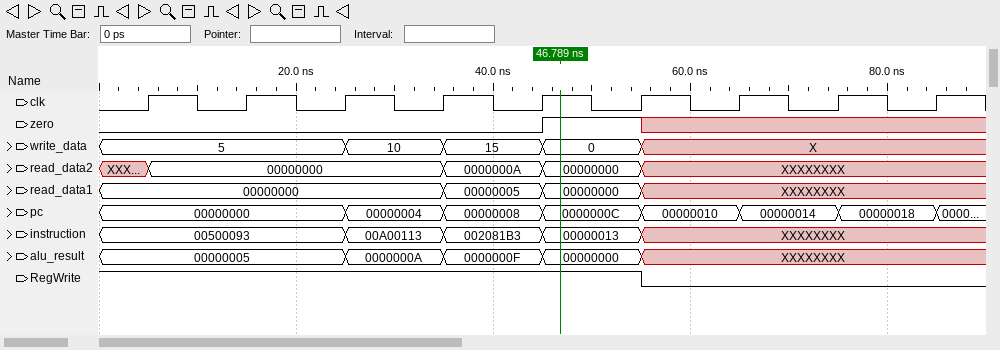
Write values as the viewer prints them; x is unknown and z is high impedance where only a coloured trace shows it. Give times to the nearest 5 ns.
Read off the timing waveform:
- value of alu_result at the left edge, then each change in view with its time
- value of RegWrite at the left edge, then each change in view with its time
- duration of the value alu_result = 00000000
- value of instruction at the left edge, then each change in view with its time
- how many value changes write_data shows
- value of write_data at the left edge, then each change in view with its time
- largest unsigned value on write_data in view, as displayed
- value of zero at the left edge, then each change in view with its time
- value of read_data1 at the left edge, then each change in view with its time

00000005, 0000000A at 25 ns, 0000000F at 35 ns, 00000000 at 45 ns, XXXXXXXX at 55 ns
1, 0 at 55 ns
10 ns
00500093, 00A00113 at 25 ns, 002081B3 at 35 ns, 00000013 at 45 ns, XXXXXXXX at 55 ns
4
5, 10 at 25 ns, 15 at 35 ns, 0 at 45 ns, X at 55 ns
15
0, 1 at 45 ns, x at 55 ns
00000000, 00000005 at 35 ns, 00000000 at 45 ns, XXXXXXXX at 55 ns
